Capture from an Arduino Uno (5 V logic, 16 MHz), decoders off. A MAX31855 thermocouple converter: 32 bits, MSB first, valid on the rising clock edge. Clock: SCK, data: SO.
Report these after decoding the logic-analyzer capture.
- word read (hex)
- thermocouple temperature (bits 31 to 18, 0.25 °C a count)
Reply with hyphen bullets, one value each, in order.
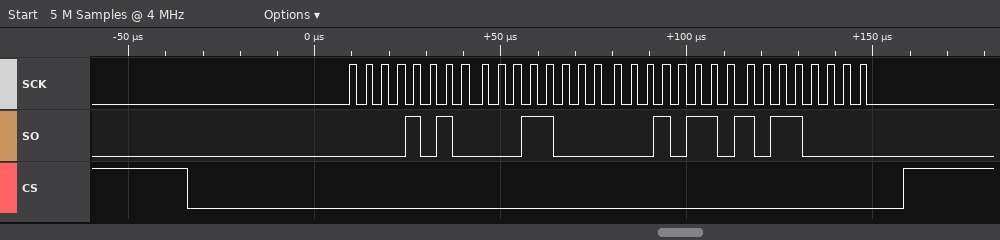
- 0x0A1816B0
- 161.50 °C
